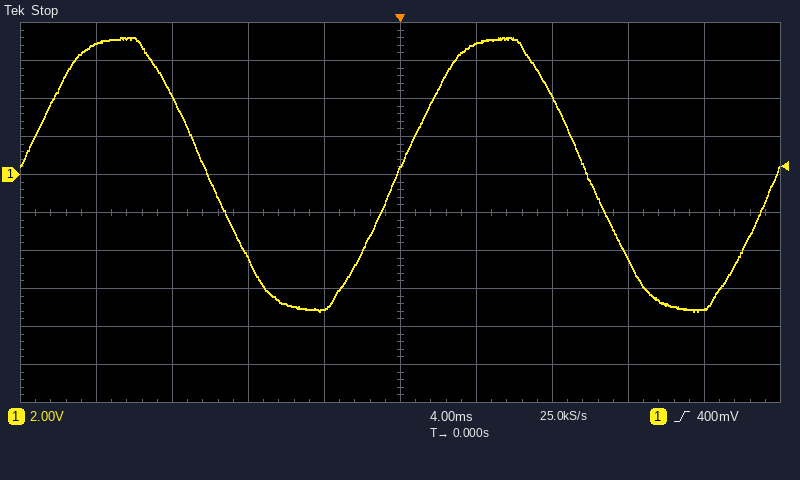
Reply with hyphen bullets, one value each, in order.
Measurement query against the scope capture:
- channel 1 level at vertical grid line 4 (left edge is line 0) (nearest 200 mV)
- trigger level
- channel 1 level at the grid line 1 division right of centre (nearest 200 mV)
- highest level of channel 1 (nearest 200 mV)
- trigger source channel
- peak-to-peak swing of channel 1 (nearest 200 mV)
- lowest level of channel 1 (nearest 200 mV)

- -7.0 V
- 400 mV
- 6.8 V
- 7.2 V
- channel 1
- 14.4 V
- -7.2 V
